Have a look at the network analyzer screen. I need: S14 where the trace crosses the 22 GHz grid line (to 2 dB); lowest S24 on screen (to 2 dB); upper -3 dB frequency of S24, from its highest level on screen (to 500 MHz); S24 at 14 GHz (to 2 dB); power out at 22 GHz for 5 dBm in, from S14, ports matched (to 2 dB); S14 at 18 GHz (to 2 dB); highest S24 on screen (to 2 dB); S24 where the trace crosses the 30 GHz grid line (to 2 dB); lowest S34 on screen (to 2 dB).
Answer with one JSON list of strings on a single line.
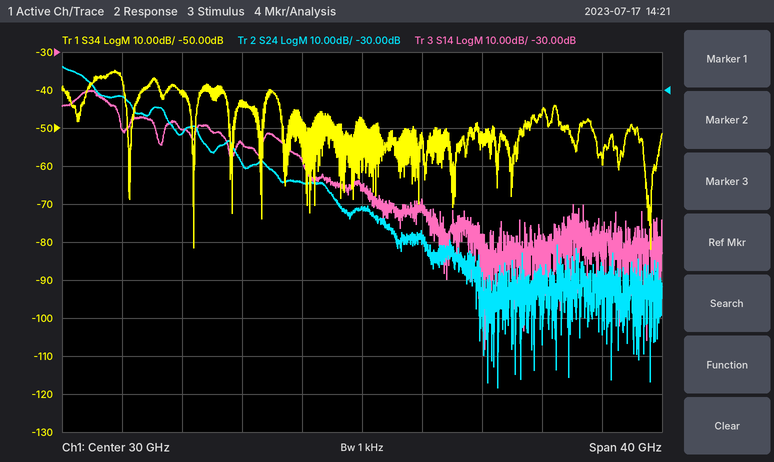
["-54 dB", "-108 dB", "11.5 GHz", "-32 dB", "-50 dBm", "-50 dB", "-24 dB", "-62 dB", "-82 dB"]
